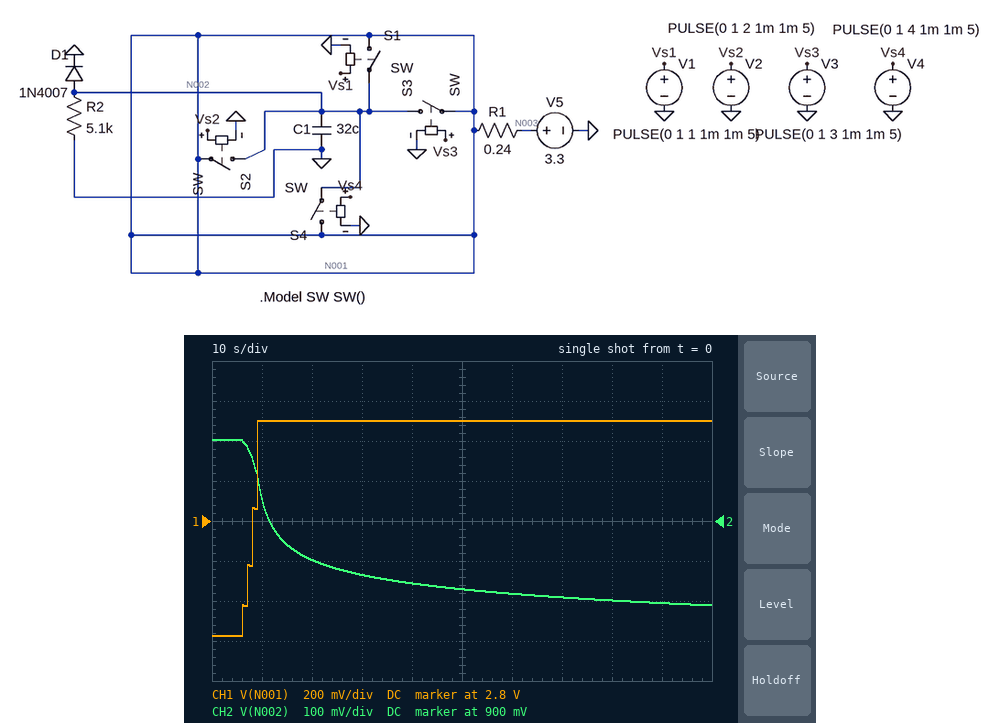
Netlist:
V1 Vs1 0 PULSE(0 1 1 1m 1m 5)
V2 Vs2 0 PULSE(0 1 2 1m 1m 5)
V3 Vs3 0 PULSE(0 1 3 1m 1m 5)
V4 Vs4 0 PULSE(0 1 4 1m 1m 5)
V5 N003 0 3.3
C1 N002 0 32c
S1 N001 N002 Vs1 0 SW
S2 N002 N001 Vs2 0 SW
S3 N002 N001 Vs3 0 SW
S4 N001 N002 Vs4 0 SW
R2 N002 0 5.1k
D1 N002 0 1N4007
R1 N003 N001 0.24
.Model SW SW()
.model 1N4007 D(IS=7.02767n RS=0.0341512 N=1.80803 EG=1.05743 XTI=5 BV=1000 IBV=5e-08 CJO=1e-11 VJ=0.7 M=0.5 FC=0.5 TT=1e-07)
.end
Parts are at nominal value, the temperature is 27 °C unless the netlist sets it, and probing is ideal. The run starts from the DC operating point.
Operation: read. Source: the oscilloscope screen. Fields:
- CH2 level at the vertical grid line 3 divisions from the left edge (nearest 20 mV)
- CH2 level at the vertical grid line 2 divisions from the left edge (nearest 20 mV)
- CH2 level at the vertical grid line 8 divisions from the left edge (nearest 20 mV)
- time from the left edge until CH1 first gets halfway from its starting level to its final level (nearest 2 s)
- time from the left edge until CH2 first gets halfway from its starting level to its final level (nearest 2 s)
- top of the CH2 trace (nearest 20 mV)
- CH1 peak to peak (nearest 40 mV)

760 mV
800 mV
700 mV
8 s
12 s
1.10 V
1.08 V
